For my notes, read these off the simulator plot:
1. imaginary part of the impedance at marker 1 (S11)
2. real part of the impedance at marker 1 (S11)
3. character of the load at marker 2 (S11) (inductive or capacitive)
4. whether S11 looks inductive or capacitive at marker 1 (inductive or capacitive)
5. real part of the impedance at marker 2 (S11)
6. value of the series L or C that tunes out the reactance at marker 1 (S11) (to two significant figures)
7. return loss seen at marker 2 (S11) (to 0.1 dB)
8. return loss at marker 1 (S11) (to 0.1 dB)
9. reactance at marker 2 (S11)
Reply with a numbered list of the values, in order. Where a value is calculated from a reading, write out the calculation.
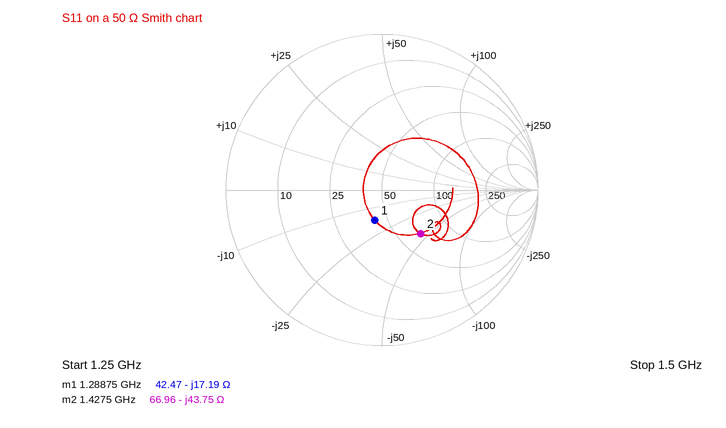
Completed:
1. -17.19 Ω
2. 42.47 Ω
3. capacitive
4. capacitive
5. 66.96 Ω
6. L = 17.19 Ω/(2π × 1.28875 GHz) ≈ 2.1 nH
7. 8.5 dB
8. 14.0 dB
9. -43.75 Ω
